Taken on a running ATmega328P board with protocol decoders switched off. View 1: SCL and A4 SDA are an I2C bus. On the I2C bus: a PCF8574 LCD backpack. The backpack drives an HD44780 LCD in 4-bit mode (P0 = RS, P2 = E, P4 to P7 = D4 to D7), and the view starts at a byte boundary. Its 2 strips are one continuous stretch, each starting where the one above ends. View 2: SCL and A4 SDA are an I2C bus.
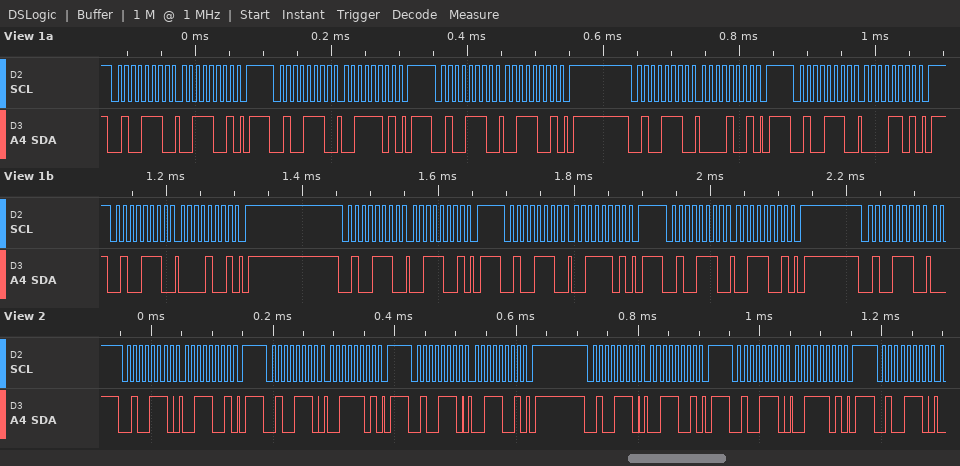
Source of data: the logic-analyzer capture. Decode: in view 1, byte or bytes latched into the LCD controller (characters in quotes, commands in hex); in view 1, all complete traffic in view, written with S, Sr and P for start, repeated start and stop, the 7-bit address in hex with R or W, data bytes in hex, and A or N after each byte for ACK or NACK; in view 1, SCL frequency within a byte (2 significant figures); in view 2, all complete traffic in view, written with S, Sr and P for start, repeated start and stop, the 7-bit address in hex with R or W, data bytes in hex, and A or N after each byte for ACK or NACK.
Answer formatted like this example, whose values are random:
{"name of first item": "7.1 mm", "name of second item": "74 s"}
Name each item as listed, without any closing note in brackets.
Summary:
{"in view 1, byte or bytes latched into the LCD controller": "'0'", "in view 1, all complete traffic in view, written with S, Sr and P for start, repeated start and stop, the 7-bit address in hex with R or W, data bytes in hex, and A or N after each byte for ACK or NACK": "S 27W A 39 A P S 27W A 3D A P S 27W A 39 A P S 27W A 09 A P S 27W A 0D A P S 27W A 09 A P S 27W A 39 A P S 27W A 3D A P S 27W A 39 A P S 27W A", "in view 1, SCL frequency within a byte": "100 kHz", "in view 2, all complete traffic in view, written with S, Sr and P for start, repeated start and stop, the 7-bit address in hex with R or W, data bytes in hex, and A or N after each byte for ACK or NACK": "S 27W A 39 A P S 27W A 3D A P S 27W A 39 A P S 27W A 39 A P S 27W A 3D A P S 27W A"}
